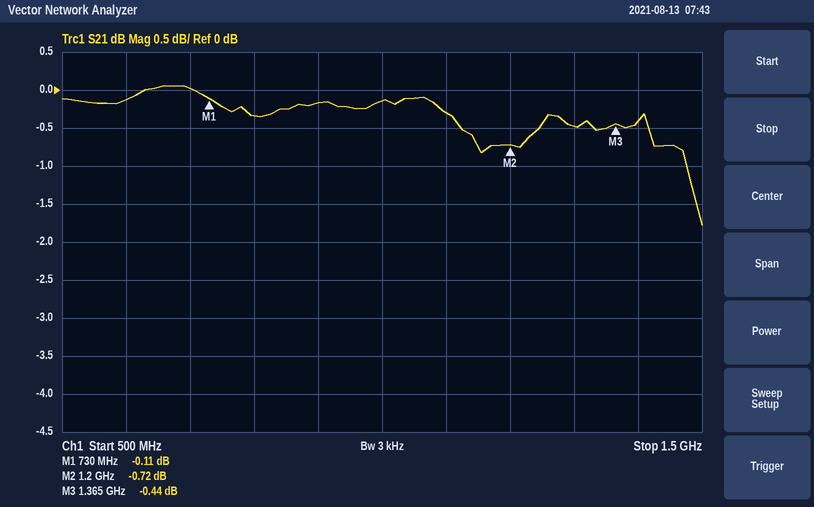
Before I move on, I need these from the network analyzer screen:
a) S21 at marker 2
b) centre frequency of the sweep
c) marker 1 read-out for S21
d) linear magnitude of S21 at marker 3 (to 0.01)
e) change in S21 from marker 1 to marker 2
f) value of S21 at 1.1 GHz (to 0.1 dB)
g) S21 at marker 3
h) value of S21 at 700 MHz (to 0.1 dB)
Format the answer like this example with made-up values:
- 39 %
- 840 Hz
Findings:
- -0.72 dB
- 1 GHz
- -0.11 dB
- 0.95
- -0.61 dB
- -0.3 dB
- -0.44 dB
- 0.0 dB
